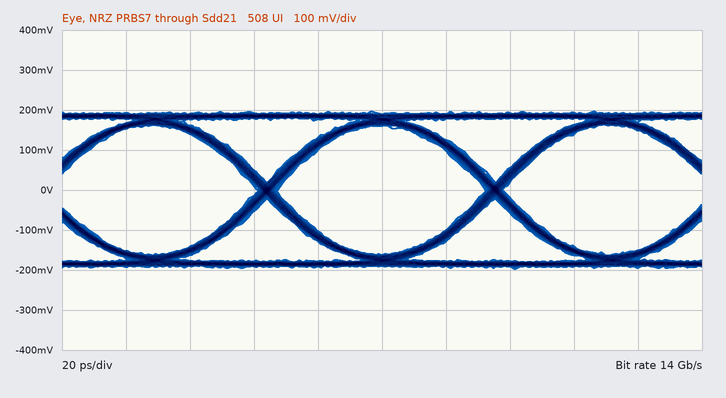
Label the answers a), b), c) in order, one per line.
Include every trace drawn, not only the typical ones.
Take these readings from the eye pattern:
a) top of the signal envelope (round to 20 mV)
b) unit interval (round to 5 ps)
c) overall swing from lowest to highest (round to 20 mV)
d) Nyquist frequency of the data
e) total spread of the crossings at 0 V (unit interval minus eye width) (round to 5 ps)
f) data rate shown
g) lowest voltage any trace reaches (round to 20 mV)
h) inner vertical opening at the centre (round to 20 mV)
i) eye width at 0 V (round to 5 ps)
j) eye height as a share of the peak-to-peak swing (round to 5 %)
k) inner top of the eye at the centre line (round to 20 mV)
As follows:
a) 200 mV
b) 70 ps
c) 400 mV
d) 7 GHz
e) 5 ps
f) 14 Gb/s
g) -200 mV
h) 320 mV
i) 65 ps
j) 80 %
k) 160 mV
